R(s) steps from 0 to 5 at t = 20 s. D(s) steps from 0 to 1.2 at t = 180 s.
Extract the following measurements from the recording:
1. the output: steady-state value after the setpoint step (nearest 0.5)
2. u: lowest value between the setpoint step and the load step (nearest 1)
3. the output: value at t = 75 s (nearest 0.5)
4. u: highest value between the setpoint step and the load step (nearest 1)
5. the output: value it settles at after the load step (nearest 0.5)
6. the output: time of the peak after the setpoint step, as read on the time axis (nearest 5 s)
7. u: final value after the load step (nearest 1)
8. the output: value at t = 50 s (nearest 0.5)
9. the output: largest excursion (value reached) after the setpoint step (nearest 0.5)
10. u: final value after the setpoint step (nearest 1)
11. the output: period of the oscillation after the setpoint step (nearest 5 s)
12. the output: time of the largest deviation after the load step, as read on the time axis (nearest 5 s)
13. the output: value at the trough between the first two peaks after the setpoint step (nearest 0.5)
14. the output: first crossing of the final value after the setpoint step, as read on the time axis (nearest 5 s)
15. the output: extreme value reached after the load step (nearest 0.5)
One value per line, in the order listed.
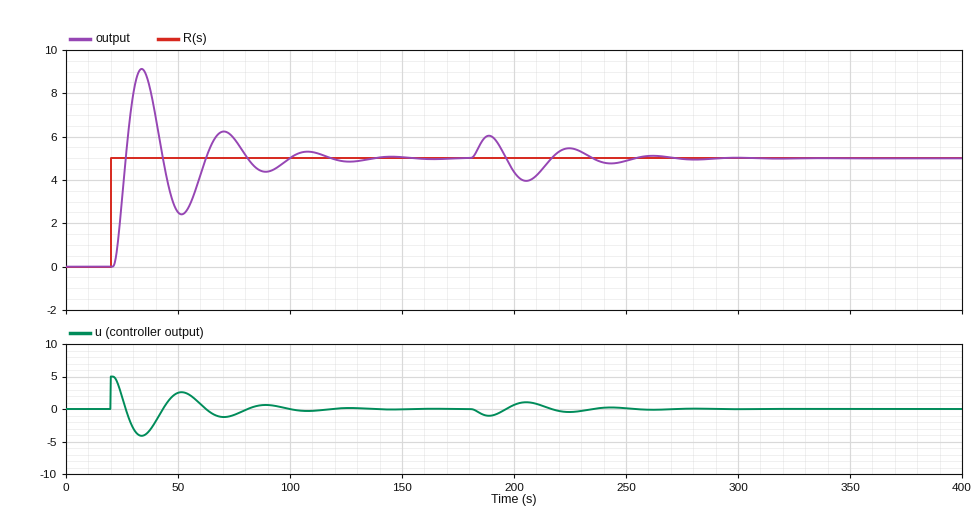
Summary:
5.0
-4
6.0
5
5.0
35 s
0
2.5
9.0
0
35 s
205 s
2.5
25 s
4.0
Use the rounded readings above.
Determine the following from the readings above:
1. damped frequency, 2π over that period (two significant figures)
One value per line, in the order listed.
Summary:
0.18 rad/s
